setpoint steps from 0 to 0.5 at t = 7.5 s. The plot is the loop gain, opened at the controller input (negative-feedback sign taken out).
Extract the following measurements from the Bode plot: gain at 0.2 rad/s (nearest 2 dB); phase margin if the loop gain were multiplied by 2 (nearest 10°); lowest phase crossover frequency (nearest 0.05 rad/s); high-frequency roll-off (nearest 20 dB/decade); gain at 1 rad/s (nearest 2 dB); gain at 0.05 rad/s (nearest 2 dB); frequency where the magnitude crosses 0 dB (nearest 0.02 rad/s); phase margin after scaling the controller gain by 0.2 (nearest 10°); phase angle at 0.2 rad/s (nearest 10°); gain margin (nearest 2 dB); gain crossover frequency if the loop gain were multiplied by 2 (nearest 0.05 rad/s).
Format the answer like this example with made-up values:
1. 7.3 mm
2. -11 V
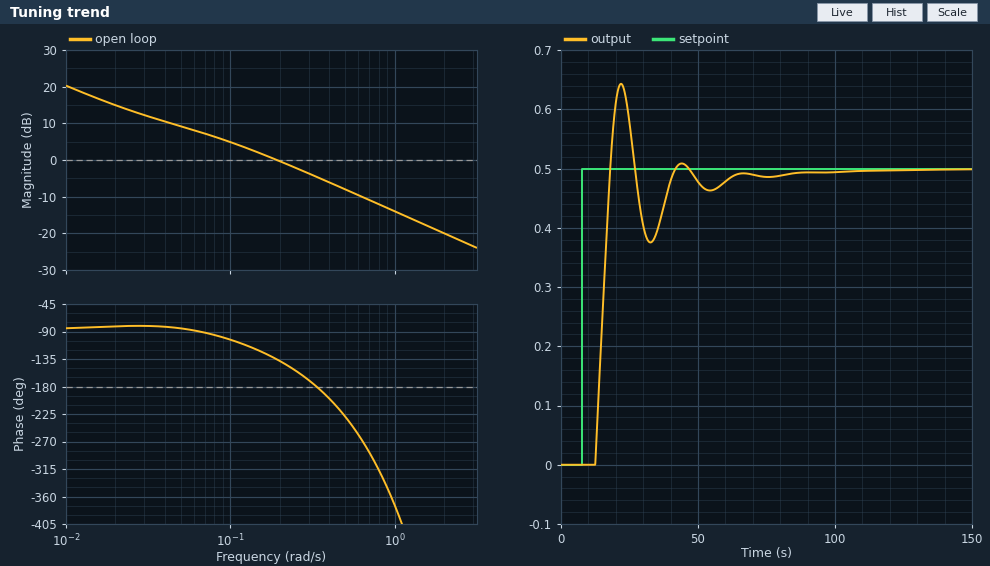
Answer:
1. 0 dB
2. -20°
3. 0.35 rad/s
4. -20 dB/decade
5. -14 dB
6. 10 dB
7. 0.20 rad/s
8. 100°
9. -140°
10. 4 dB
11. 0.40 rad/s
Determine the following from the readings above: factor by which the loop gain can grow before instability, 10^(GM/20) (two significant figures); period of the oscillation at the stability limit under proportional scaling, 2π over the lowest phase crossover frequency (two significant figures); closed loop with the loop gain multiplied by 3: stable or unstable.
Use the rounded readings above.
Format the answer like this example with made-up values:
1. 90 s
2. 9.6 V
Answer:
1. 1.6
2. 18 s
3. unstable
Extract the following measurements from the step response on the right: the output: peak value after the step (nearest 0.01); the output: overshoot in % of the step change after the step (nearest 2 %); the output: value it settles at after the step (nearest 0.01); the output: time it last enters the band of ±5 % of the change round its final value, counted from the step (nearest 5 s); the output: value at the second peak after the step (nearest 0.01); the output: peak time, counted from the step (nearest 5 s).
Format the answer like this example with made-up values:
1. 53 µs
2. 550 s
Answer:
1. 0.64
2. 28 %
3. 0.50
4. 50 s
5. 0.51
6. 15 s
